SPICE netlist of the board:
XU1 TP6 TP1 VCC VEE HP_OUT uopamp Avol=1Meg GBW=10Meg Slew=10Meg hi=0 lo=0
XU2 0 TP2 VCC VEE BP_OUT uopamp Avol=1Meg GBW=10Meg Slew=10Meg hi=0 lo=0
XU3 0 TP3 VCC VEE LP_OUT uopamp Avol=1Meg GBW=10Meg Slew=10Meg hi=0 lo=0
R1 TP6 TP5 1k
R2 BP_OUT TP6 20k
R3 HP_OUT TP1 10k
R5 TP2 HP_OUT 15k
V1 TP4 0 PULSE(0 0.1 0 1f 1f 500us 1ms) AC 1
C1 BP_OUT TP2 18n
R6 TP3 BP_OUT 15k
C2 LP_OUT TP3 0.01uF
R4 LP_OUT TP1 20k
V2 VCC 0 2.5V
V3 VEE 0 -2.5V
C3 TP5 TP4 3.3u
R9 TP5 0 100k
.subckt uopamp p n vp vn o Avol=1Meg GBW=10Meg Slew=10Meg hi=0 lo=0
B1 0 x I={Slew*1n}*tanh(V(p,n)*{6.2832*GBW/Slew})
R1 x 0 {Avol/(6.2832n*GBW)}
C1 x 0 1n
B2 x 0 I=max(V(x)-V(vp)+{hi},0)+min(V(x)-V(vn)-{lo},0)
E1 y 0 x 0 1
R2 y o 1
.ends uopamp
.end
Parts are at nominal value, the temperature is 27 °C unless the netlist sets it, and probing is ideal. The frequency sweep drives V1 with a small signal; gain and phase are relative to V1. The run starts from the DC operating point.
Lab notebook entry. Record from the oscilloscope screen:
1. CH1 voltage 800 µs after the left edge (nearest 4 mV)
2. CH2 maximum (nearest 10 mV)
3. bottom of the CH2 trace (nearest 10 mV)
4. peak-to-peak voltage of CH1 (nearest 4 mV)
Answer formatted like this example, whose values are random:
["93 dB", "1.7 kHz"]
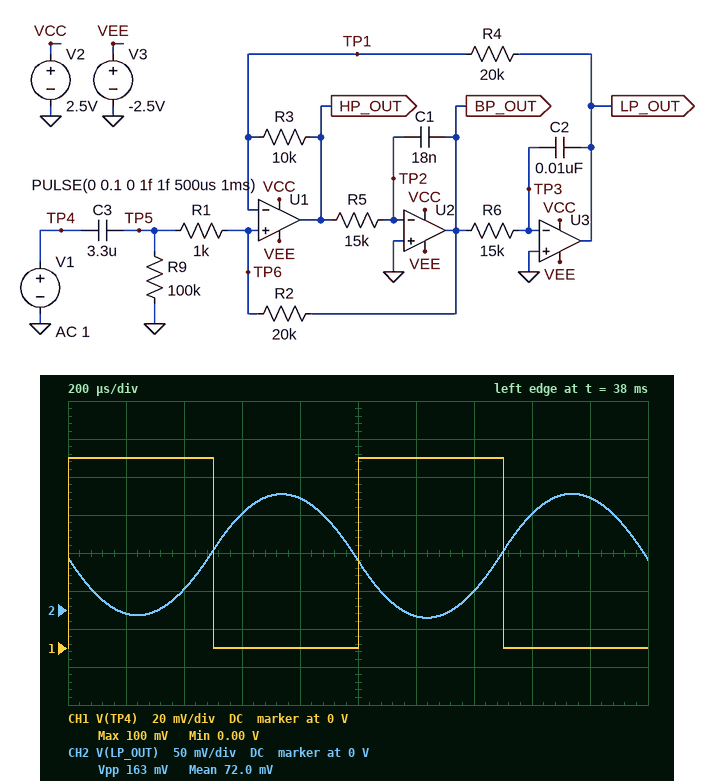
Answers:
["0 V", "150 mV", "-10 mV", "100 mV"]
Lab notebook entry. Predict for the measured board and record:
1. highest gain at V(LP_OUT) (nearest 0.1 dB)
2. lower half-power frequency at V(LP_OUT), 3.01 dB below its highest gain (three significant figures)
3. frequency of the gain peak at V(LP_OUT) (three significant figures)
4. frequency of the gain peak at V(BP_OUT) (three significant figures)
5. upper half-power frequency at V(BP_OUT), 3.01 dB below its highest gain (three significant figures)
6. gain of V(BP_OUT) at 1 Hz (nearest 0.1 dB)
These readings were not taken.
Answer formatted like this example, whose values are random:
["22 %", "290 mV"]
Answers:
["31.6 dB", "539 Hz", "560 Hz", "561 Hz", "582 Hz", "-60.8 dB"]
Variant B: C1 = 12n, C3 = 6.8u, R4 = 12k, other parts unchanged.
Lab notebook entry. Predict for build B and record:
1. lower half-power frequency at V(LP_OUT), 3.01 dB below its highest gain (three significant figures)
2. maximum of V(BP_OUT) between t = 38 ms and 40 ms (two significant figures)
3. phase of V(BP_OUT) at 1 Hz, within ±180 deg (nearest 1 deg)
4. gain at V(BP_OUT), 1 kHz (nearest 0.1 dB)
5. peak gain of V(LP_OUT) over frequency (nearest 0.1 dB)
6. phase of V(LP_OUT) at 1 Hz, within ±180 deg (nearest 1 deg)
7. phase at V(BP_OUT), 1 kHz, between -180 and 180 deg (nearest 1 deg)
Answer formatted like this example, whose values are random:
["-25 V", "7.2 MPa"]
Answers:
["844 Hz", "430 mV", "-37 deg", "16.5 dB", "27.6 dB", "53 deg", "110 deg"]
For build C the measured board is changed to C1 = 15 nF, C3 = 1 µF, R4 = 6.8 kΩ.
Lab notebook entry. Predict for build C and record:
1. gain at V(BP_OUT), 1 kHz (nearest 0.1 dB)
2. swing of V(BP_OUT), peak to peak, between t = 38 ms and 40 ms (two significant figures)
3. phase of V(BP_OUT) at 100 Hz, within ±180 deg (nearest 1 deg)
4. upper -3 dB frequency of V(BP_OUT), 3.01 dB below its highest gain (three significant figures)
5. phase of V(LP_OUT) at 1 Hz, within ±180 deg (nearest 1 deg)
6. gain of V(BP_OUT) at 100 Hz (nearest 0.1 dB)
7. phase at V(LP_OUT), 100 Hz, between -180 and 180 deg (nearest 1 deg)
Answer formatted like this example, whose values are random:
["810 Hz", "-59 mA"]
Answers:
["21.3 dB", "1.5 V", "-85 deg", "1.10 kHz", "84 deg", "-16.5 dB", "5 deg"]
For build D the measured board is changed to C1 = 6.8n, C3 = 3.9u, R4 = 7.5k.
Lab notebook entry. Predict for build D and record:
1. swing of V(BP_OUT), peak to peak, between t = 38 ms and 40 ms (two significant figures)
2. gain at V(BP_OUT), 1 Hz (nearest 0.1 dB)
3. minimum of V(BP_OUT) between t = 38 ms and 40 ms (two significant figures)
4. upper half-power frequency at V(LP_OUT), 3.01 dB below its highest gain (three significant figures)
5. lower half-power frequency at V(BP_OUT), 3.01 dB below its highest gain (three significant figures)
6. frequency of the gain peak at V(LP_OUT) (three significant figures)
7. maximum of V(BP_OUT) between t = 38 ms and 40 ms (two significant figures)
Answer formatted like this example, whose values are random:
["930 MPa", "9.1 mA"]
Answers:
["360 mV", "-64.2 dB", "-180 mV", "1.57 kHz", "1.40 kHz", "1.48 kHz", "180 mV"]
